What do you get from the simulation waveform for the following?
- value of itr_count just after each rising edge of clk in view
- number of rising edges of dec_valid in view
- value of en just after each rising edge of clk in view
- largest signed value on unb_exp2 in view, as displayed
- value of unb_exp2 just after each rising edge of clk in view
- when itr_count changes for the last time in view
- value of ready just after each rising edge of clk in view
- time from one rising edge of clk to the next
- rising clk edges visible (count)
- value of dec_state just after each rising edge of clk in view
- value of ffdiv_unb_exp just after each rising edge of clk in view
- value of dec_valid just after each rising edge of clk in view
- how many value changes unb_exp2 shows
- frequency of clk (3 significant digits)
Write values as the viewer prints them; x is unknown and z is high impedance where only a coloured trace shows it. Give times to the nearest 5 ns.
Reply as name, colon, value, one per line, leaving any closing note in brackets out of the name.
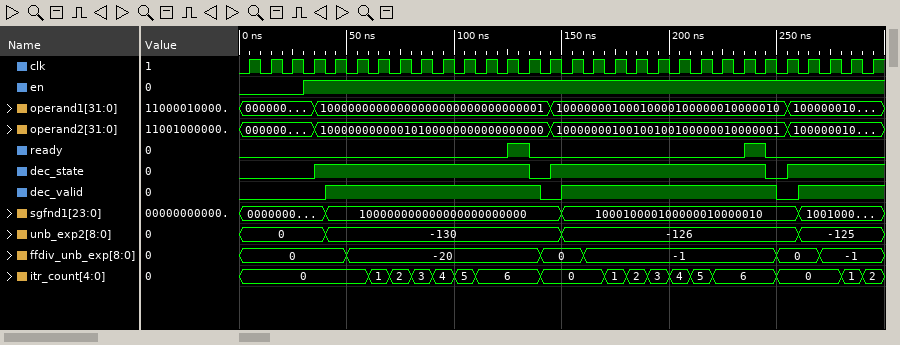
value of itr_count just after each rising edge of clk in view: 0, 0, 0, 0, 0, 0, 1, 2, 3, 4, 5, 6, 6, 6, 0, 0, 0, 1, 2, 3, 4, 5, 6, 6, 6, 0, 0, 0, 1, 2
number of rising edges of dec_valid in view: 3
value of en just after each rising edge of clk in view: 0 0 0 1 1 1 1 1 1 1 1 1 1 1 1 1 1 1 1 1 1 1 1 1 1 1 1 1 1 1
largest signed value on unb_exp2 in view, as displayed: 0
value of unb_exp2 just after each rising edge of clk in view: 0, 0, 0, 0, -130, -130, -130, -130, -130, -130, -130, -130, -130, -130, -130, -126, -126, -126, -126, -126, -126, -126, -126, -126, -126, -126, -125, -125, -125, -125
when itr_count changes for the last time in view: 290 ns
value of ready just after each rising edge of clk in view: 0 0 0 0 0 0 0 0 0 0 0 0 1 0 0 0 0 0 0 0 0 0 0 1 0 0 0 0 0 0
time from one rising edge of clk to the next: 10 ns
rising clk edges visible: 30
value of dec_state just after each rising edge of clk in view: 0 0 0 1 1 1 1 1 1 1 1 1 1 0 1 1 1 1 1 1 1 1 1 1 0 1 1 1 1 1
value of ffdiv_unb_exp just after each rising edge of clk in view: 0, 0, 0, 0, 0, -20, -20, -20, -20, -20, -20, -20, -20, -20, 0, 0, -1, -1, -1, -1, -1, -1, -1, -1, -1, 0, 0, -1, -1, -1
value of dec_valid just after each rising edge of clk in view: 0 0 0 0 1 1 1 1 1 1 1 1 1 1 0 1 1 1 1 1 1 1 1 1 1 0 1 1 1 1
how many value changes unb_exp2 shows: 3
frequency of clk: 100 MHz
